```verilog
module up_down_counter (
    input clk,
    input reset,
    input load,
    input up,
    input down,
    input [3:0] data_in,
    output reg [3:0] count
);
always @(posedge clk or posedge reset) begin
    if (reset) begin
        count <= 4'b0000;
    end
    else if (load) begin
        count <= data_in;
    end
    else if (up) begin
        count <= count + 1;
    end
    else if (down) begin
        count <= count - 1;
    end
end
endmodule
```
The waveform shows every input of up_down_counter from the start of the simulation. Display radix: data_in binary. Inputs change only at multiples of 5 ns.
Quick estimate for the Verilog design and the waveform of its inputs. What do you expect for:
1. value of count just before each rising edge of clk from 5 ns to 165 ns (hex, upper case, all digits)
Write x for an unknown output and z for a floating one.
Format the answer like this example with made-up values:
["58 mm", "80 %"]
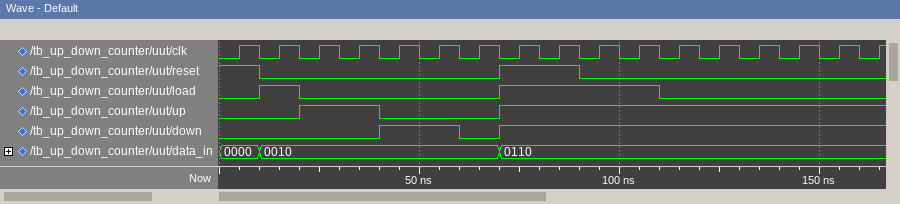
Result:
["0, 0, 2, 3, 4, 3, 2, 0, 0, 0, 6, 6, 7, 8, 9, A, B"]
